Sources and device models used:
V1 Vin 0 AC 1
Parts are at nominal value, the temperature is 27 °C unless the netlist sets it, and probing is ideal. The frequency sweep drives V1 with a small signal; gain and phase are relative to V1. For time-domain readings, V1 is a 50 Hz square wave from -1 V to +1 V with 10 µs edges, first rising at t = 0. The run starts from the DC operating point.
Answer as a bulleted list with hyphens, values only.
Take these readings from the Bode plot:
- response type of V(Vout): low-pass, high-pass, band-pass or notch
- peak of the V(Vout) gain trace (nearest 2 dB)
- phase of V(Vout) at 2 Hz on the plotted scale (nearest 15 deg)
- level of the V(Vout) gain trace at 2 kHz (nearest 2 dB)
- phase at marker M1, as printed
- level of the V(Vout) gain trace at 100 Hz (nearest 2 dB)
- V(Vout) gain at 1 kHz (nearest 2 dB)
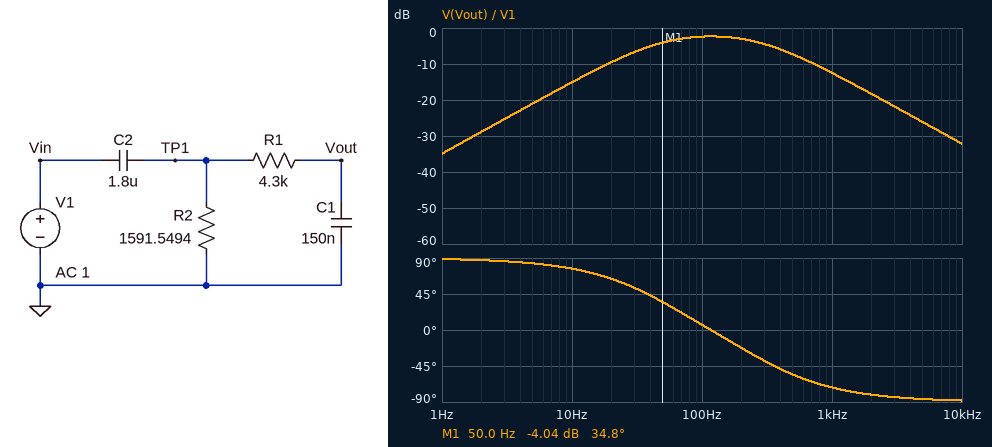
- band-pass
- -2 dB
- 90 deg
- -18 dB
- 34.8 deg
- -2 dB
- -12 dB
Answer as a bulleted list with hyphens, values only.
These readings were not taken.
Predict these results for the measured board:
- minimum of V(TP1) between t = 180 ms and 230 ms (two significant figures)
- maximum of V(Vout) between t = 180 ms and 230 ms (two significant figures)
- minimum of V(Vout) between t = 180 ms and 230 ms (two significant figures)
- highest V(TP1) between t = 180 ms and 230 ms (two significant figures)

- -1.9 V
- 1.2 V
- -1.2 V
- 1.9 V
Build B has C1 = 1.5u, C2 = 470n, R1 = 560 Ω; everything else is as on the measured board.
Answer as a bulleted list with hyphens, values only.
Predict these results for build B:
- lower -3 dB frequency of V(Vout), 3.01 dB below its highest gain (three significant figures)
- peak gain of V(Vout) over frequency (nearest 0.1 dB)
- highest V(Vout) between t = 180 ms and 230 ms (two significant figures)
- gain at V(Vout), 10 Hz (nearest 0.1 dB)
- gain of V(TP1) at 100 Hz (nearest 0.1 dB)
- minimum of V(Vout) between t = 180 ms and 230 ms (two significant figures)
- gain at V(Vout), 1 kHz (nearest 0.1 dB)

- 38.6 Hz
- -14.5 dB
- 320 mV
- -26.8 dB
- -13.8 dB
- -320 mV
- -17.3 dB
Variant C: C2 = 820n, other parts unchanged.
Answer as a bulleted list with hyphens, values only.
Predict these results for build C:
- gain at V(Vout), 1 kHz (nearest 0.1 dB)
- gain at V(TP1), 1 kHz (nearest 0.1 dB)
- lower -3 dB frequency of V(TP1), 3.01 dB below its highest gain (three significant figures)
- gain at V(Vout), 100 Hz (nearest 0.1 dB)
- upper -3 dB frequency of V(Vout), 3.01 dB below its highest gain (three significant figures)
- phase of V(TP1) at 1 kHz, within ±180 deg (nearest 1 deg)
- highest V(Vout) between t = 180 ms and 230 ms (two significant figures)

- -12.6 dB
- -0.2 dB
- 159 Hz
- -5.4 dB
- 477 Hz
- 9 deg
- 920 mV
